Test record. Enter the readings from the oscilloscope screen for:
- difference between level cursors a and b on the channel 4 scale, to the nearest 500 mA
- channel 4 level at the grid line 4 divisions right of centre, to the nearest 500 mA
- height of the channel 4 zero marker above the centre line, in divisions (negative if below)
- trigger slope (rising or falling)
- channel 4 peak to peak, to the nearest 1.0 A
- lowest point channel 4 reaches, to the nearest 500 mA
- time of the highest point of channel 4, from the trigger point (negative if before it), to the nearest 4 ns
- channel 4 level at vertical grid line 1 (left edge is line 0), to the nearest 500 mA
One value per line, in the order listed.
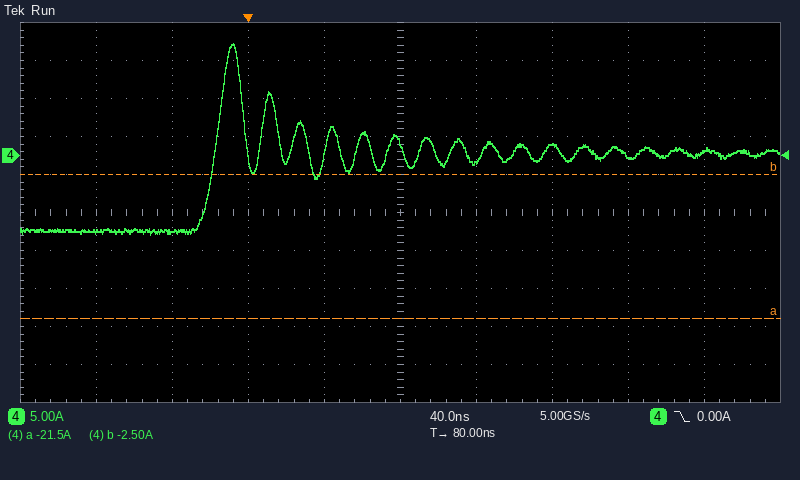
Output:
19.0 A
500 mA
+1.5 div
falling
25.0 A
-10.5 A
-8 ns
-10.0 A
